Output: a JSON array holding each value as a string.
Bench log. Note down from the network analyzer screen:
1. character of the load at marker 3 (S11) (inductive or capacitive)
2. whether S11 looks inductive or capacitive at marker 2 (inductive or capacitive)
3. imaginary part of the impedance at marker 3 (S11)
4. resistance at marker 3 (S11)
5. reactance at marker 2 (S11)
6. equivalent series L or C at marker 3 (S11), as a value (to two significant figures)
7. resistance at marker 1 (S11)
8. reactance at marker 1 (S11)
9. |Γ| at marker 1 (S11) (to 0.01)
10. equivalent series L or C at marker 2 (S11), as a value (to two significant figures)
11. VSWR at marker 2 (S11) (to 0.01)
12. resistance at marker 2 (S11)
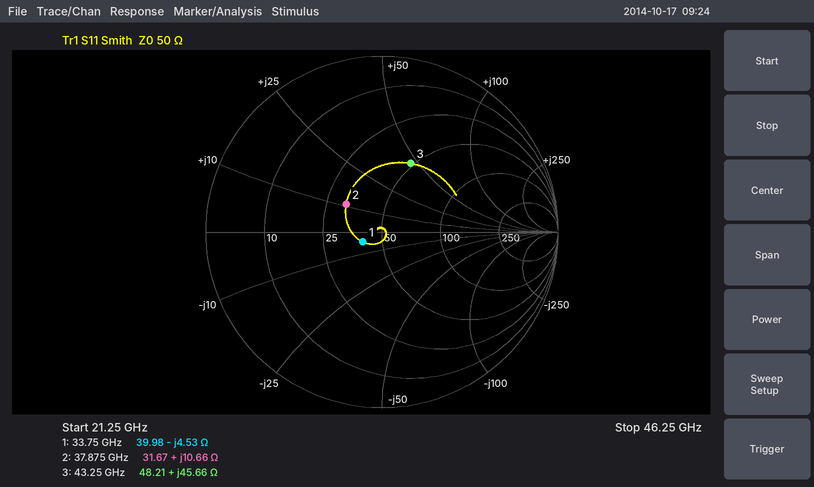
["inductive", "inductive", "+45.66 Ω", "48.21 Ω", "+10.66 Ω", "170 pH", "39.98 Ω", "-4.53 Ω", "0.12", "45 pH", "1.69", "31.67 Ω"]
